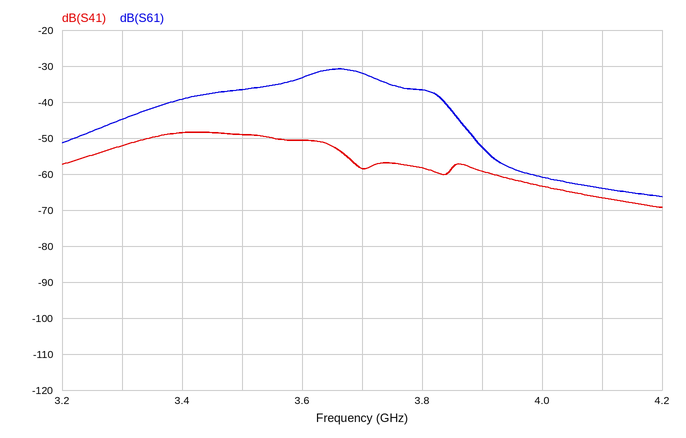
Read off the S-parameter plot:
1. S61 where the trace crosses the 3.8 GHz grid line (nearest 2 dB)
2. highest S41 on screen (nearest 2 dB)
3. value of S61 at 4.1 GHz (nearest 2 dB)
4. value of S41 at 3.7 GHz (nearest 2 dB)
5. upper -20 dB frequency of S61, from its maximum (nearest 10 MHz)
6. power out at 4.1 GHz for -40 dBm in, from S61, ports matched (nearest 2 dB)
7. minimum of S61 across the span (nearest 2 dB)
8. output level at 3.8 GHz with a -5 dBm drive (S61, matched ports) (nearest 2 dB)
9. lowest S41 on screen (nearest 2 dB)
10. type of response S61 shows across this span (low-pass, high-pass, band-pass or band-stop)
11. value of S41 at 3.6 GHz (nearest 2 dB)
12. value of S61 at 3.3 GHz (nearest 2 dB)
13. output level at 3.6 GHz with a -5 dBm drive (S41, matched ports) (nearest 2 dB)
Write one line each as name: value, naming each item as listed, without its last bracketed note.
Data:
S61 where the trace crosses the 3.8 GHz grid line: -36 dB
highest S41 on screen: -48 dB
value of S61 at 4.1 GHz: -64 dB
value of S41 at 3.7 GHz: -58 dB
upper -20 dB frequency of S61, from its maximum: 3.89 GHz
power out at 4.1 GHz for -40 dBm in, from S61, ports matched: -104 dBm
minimum of S61 across the span: -66 dB
output level at 3.8 GHz with a -5 dBm drive (S61, matched ports): -42 dBm
lowest S41 on screen: -70 dB
type of response S61 shows across this span: band-pass
value of S41 at 3.6 GHz: -50 dB
value of S61 at 3.3 GHz: -44 dB
output level at 3.6 GHz with a -5 dBm drive (S41, matched ports): -56 dBm
